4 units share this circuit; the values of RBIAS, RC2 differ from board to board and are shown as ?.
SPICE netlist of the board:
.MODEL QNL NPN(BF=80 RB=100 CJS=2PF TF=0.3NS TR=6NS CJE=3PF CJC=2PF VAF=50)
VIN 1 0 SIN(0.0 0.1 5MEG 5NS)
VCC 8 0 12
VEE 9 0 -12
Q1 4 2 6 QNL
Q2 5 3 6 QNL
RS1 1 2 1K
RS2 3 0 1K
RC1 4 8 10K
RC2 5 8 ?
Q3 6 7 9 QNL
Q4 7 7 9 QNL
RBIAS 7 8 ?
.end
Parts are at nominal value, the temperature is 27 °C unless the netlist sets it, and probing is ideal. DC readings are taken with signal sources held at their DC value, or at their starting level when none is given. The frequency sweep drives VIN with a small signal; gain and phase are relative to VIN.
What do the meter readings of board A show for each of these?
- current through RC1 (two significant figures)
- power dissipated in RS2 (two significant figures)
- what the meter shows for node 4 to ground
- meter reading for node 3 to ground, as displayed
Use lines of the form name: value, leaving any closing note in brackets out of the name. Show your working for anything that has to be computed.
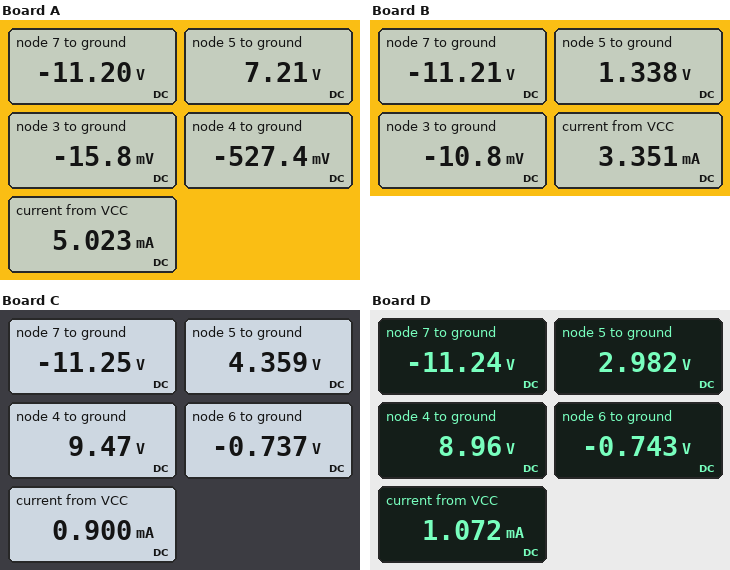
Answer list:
current through RC1: (12 V - (-527.4 mV)) / 10 kΩ = 1.3 mA
power dissipated in RS2: (0 V - (-15.8 mV))^2 / 1 kΩ = 250 nW
what the meter shows for node 4 to ground: -527.4 mV
meter reading for node 3 to ground, as displayed: -15.8 mV
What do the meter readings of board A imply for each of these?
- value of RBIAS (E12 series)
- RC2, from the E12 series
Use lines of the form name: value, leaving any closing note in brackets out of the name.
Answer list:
value of RBIAS: 10 kΩ
RC2, from the E12 series: 3.3 kΩ
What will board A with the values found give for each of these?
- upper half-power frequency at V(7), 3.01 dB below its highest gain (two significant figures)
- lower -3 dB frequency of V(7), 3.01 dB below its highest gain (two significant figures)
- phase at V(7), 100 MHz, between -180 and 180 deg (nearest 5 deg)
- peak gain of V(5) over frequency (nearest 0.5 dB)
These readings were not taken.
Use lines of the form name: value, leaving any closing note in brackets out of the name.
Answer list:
upper half-power frequency at V(7), 3.01 dB below its highest gain: 360 MHz
lower -3 dB frequency of V(7), 3.01 dB below its highest gain: 64 MHz
phase at V(7), 100 MHz, between -180 and 180 deg: 15 deg
peak gain of V(5) over frequency: 31.0 dB
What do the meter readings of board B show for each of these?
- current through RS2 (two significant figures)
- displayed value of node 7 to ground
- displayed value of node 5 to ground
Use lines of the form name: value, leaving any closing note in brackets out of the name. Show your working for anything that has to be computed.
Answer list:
current through RS2: (0 V - (-10.8 mV)) / 1 kΩ = 11 µA
displayed value of node 7 to ground: -11.21 V
displayed value of node 5 to ground: 1.338 V
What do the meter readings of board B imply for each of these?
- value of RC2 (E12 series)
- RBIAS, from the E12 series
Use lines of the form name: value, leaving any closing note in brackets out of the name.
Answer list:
value of RC2: 12 kΩ
RBIAS, from the E12 series: 15 kΩ
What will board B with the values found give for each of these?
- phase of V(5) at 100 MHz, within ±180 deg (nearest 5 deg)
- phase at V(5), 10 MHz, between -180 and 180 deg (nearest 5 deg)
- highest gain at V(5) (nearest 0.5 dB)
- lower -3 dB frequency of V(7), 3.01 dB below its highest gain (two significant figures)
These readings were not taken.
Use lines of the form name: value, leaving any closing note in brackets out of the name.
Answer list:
phase of V(5) at 100 MHz, within ±180 deg: -120 deg
phase at V(5), 10 MHz, between -180 and 180 deg: -100 deg
highest gain at V(5): 41.5 dB
lower -3 dB frequency of V(7), 3.01 dB below its highest gain: 46 MHz
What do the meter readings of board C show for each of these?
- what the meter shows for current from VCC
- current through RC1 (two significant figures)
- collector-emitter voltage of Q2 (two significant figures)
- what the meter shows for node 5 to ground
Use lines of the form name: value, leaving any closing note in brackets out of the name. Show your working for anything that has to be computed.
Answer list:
what the meter shows for current from VCC: 0.900 mA
current through RC1: (12 V - 9.47 V) / 10 kΩ = 250 µA
collector-emitter voltage of Q2: 4.359 V - (-737 mV) = 5.1 V
what the meter shows for node 5 to ground: 4.359 V
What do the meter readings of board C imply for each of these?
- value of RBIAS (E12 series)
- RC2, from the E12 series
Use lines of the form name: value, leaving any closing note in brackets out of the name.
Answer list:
value of RBIAS: 56 kΩ
RC2, from the E12 series: 33 kΩ
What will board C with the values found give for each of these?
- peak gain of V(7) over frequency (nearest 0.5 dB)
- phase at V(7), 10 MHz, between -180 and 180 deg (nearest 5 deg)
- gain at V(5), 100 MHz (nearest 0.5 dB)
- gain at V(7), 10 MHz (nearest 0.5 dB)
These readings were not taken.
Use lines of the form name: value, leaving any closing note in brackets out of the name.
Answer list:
peak gain of V(7) over frequency: -42.5 dB
phase at V(7), 10 MHz, between -180 and 180 deg: 70 deg
gain at V(5), 100 MHz: -14.0 dB
gain at V(7), 10 MHz: -55.0 dB
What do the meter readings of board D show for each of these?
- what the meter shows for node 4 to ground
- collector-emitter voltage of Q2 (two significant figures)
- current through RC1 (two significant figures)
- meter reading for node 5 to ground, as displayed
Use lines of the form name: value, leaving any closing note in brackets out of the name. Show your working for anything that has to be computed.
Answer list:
what the meter shows for node 4 to ground: 8.96 V
collector-emitter voltage of Q2: 2.982 V - (-743 mV) = 3.7 V
current through RC1: (12 V - 8.96 V) / 10 kΩ = 300 µA
meter reading for node 5 to ground, as displayed: 2.982 V
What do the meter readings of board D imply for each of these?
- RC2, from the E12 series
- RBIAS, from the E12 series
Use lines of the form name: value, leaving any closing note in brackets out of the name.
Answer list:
RC2, from the E12 series: 33 kΩ
RBIAS, from the E12 series: 47 kΩ
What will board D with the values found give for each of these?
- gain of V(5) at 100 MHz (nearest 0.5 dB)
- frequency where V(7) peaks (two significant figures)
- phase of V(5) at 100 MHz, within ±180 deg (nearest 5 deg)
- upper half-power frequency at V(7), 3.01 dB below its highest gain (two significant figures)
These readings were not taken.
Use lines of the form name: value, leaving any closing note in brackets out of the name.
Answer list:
gain of V(5) at 100 MHz: -13.5 dB
frequency where V(7) peaks: 89 MHz
phase of V(5) at 100 MHz, within ±180 deg: -140 deg
upper half-power frequency at V(7), 3.01 dB below its highest gain: 210 MHz
